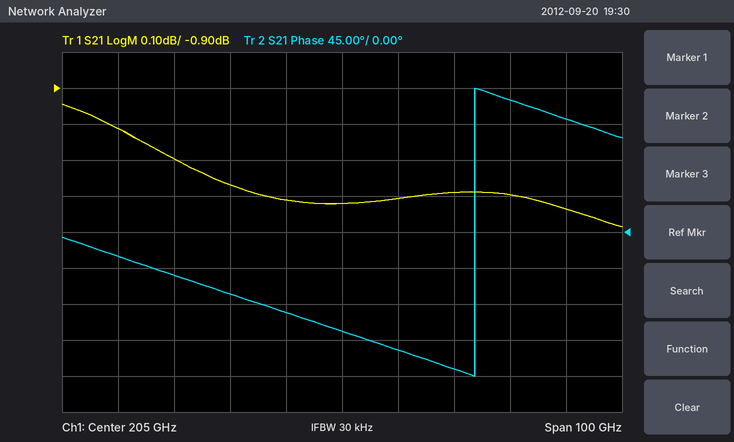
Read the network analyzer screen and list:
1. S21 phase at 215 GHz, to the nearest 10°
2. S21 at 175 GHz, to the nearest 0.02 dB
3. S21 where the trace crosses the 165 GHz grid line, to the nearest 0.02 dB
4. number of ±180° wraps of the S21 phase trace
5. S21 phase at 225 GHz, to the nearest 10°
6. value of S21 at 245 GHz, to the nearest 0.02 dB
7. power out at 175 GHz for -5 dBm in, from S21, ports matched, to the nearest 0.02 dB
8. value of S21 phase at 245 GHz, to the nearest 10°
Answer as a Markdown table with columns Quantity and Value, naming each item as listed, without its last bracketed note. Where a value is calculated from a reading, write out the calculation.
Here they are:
| Quantity | Value |
|---|---|
| S21 phase at 215 GHz, to the nearest 10° | -150° |
| S21 at 175 GHz, to the nearest 0.02 dB | -1.10 dB |
| S21 where the trace crosses the 165 GHz grid line, to the nearest 0.02 dB | -1.02 dB |
| number of ±180° wraps of the S21 phase trace | 1 |
| S21 phase at 225 GHz, to the nearest 10° | -170° |
| value of S21 at 245 GHz, to the nearest 0.02 dB | -1.24 dB |
| power out at 175 GHz for -5 dBm in, from S21, ports matched, to the nearest 0.02 dB | -5 dBm + (-1.10 dB) = -6.10 dBm |
| value of S21 phase at 245 GHz, to the nearest 10° | 140° |
